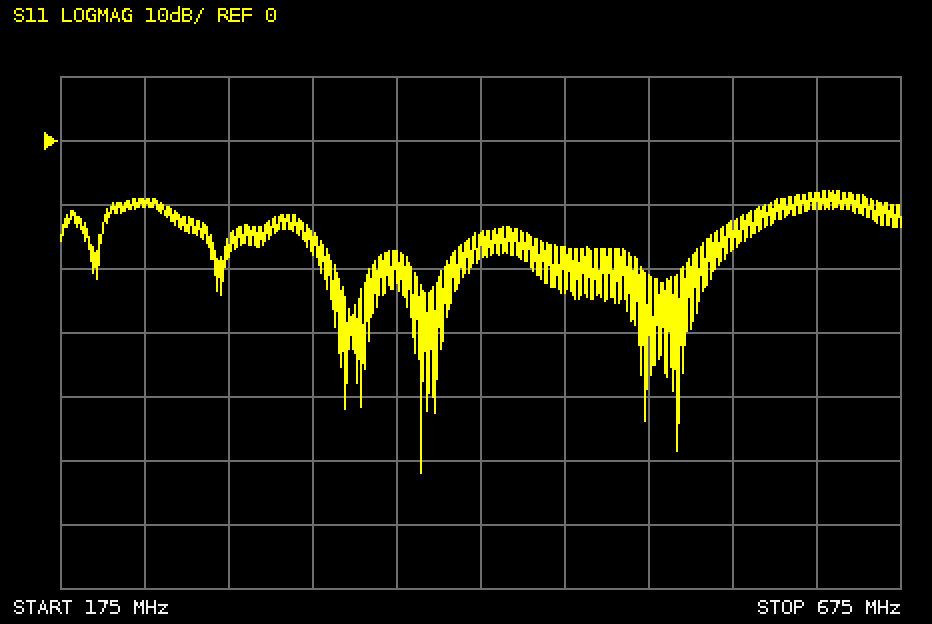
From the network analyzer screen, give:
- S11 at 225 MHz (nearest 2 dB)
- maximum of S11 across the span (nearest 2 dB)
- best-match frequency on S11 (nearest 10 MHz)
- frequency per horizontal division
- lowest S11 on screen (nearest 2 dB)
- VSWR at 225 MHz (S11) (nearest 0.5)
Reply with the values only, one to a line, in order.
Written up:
-10 dB
-8 dB
390 MHz
50 MHz
-52 dB
2.0
